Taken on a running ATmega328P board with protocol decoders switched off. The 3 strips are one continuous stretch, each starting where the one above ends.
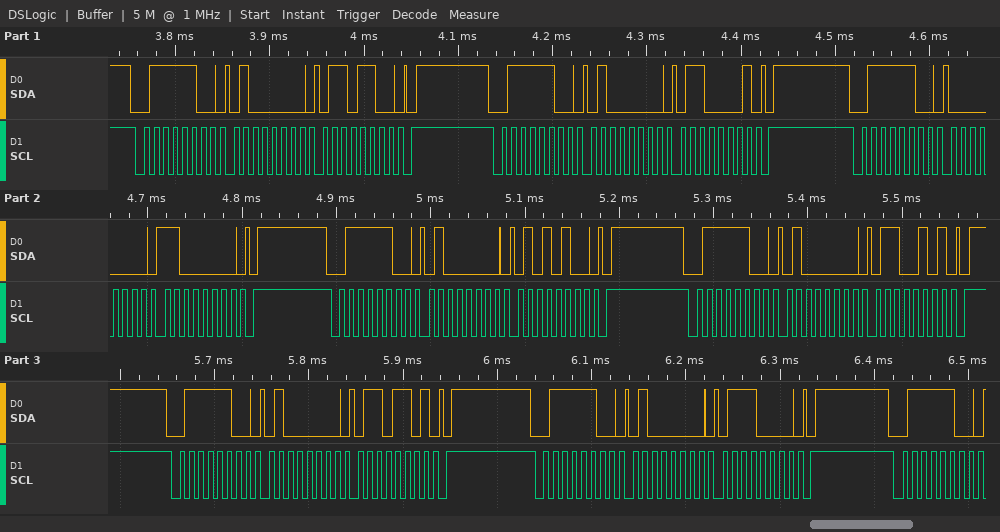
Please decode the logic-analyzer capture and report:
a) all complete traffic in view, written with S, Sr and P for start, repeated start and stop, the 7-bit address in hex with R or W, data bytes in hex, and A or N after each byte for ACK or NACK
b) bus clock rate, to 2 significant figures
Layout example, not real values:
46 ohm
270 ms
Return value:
S 3EW A 40 A 6C A P S 3EW A 40 A 61 A P S 3EW A 00 A C0 A P S 3EW A 40 A 54 A P S 3EW A 40 A 65 A P S 3EW A 40 A 6D A P S 3EW A 40 A 70 A P S 3EW A
100 kHz
